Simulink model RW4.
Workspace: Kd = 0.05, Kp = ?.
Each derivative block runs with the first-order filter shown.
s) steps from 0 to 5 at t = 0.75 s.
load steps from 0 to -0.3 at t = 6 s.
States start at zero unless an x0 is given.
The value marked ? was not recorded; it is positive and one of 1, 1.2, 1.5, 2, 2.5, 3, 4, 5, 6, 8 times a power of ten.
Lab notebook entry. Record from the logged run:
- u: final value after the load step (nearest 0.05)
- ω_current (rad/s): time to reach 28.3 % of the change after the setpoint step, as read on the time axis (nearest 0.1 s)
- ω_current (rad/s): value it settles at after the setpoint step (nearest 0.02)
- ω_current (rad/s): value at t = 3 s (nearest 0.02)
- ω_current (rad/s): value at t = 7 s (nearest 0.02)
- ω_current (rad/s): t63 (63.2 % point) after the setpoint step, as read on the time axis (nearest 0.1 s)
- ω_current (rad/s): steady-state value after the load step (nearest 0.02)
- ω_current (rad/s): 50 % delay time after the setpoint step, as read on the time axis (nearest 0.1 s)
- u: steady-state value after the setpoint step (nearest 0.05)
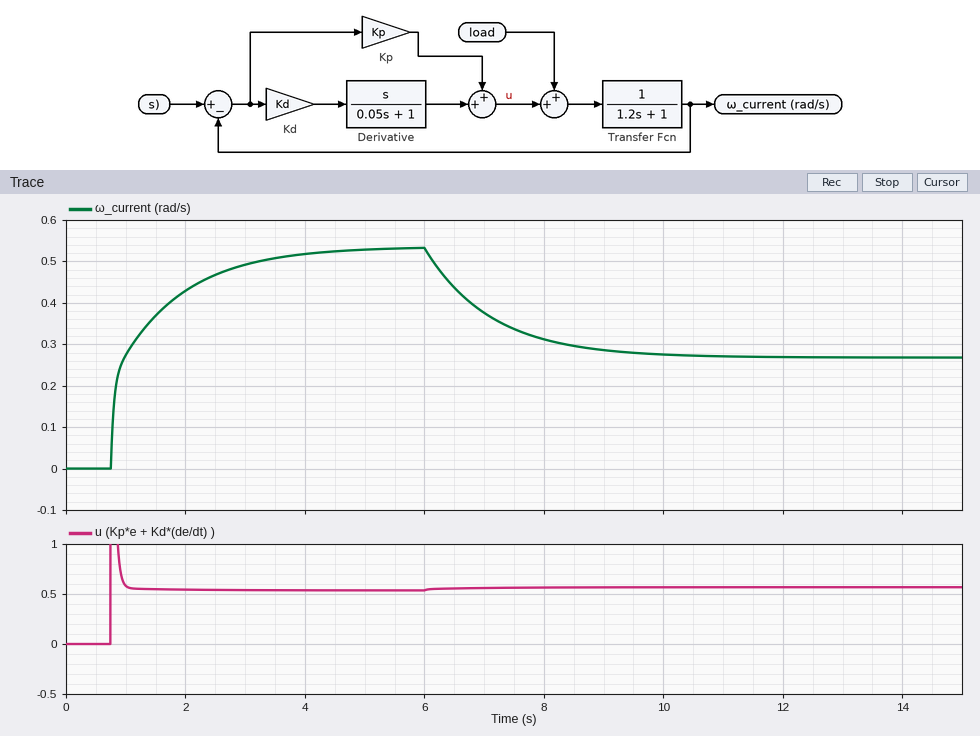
0.55
0.8 s
0.54
0.50
0.38
1.3 s
0.26
1.0 s
0.55
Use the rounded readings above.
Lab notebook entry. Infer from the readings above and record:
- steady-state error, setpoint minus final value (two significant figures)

4.5
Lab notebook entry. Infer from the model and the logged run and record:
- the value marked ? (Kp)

0.12
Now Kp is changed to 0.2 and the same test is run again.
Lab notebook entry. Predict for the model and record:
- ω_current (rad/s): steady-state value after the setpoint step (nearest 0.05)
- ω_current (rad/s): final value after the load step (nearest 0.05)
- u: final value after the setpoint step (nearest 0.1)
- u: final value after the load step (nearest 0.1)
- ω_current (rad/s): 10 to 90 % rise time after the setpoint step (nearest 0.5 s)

0.85
0.60
0.8
0.9
2.0 s
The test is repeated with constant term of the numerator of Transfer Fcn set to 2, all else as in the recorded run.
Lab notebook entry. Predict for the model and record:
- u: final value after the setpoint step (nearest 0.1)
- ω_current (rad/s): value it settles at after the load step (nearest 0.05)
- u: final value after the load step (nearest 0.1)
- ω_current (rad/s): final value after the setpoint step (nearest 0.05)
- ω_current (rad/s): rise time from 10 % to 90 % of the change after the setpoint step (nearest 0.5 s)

0.5
0.50
0.5
0.95
2.0 s
